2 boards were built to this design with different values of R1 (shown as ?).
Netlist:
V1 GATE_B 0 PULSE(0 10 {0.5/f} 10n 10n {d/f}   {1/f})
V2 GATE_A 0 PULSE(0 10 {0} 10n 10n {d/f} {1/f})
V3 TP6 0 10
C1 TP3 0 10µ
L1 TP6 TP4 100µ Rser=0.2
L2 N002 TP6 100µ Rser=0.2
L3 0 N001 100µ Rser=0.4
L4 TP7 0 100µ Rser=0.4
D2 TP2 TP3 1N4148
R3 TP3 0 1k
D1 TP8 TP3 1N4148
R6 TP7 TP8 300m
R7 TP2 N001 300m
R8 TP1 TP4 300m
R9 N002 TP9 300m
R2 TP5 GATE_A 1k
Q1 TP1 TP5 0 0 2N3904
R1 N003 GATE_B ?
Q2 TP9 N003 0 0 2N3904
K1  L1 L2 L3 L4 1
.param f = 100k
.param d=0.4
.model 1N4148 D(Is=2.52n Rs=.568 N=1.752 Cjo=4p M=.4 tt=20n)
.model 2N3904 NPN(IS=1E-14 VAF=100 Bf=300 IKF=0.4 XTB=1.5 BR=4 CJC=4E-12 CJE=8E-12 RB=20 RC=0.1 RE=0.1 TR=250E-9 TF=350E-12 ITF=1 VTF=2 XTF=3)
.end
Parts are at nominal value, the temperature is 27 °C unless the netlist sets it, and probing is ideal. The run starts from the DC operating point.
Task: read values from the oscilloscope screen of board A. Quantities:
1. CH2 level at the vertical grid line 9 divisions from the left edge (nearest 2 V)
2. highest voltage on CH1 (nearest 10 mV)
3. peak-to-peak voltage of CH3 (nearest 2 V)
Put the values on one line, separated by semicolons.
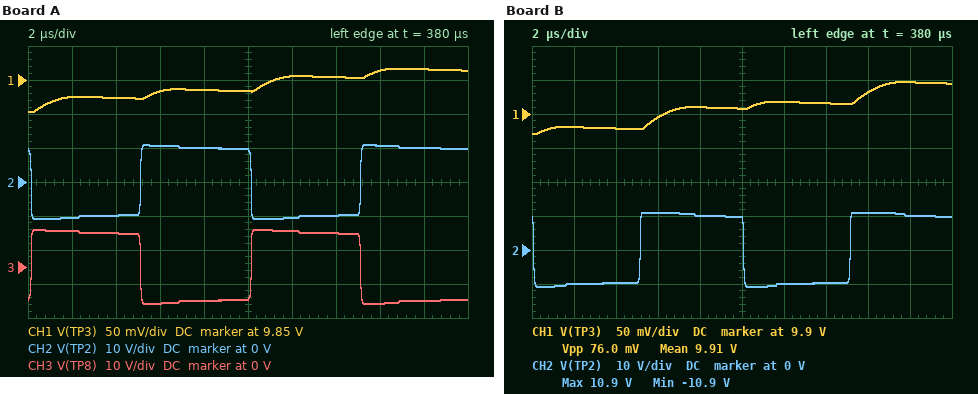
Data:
10 V; 9.87 V; 22 V
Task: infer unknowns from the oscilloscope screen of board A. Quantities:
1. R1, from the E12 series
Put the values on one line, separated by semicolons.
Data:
820 Ω
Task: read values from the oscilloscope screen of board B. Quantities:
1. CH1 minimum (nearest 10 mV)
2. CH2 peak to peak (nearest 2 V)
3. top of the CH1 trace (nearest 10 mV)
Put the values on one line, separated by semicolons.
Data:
9.87 V; 22 V; 9.95 V
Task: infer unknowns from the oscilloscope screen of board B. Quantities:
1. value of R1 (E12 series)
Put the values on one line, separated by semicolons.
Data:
1.8 kΩ
